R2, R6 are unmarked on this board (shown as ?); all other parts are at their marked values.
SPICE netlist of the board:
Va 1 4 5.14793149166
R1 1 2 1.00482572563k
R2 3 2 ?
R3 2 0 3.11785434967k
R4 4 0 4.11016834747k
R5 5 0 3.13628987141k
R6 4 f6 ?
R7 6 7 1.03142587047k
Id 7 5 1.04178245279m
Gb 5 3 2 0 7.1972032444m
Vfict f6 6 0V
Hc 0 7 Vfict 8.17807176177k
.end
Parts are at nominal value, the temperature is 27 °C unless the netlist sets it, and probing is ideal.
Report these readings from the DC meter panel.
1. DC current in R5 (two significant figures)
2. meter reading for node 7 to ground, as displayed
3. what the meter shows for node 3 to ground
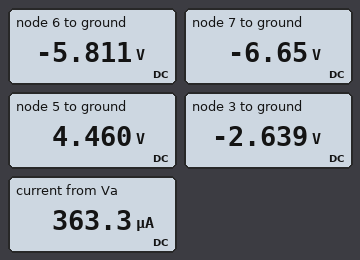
1.4 mA
-6.65 V
-2.639 V
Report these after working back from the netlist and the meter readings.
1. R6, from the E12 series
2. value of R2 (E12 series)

1.2 kΩ
6.8 kΩ
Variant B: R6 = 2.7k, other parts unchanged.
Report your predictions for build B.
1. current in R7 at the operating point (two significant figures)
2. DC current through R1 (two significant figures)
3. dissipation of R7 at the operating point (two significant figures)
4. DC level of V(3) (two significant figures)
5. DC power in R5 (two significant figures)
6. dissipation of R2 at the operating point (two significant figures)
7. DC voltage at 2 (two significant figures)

1.1 mA
93 µA
1.3 mW
-680 mV
4.1 mW
65 µW
-14 mV
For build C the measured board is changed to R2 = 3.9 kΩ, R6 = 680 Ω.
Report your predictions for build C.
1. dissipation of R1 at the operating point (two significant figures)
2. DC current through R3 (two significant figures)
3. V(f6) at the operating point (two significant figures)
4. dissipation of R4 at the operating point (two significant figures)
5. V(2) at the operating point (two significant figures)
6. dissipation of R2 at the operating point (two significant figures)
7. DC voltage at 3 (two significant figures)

180 µW
20 µA
-5.3 V
5.6 mW
-62 mV
770 µW
-1.8 V
